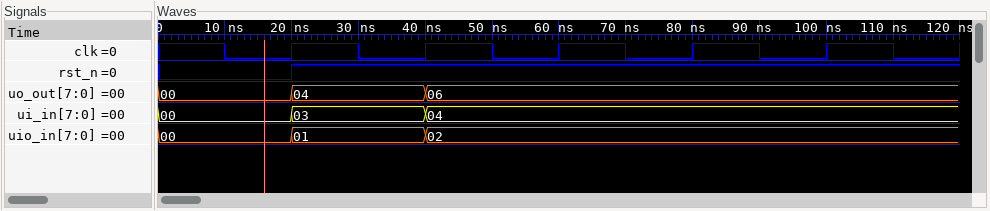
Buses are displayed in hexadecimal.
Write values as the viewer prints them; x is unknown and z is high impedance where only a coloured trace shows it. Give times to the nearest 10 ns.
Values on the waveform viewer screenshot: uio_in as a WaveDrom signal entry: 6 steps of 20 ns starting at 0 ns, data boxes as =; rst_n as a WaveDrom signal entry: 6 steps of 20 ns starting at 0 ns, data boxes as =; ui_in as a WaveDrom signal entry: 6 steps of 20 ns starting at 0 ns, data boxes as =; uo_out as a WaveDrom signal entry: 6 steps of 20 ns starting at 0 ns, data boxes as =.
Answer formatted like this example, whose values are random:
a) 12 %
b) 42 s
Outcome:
a) {name: 'uio_in', wave: '===...', data: '00 01 02'}
b) {name: 'rst_n', wave: '01....'}
c) {name: 'ui_in', wave: '===...', data: '00 03 04'}
d) {name: 'uo_out', wave: '===...', data: '00 04 06'}
